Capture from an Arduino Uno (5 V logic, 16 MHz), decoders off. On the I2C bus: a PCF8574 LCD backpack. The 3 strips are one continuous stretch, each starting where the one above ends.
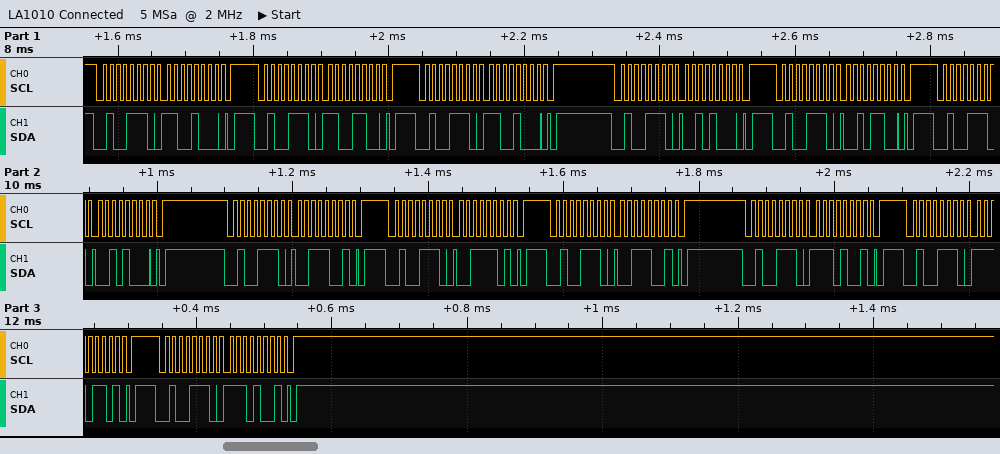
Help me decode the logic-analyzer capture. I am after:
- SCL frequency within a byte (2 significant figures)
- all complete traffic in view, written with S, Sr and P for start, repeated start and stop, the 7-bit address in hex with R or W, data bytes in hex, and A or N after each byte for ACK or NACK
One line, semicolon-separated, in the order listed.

100 kHz; S 27W A C8 A P S 27W A CC A P S 27W A C8 A P S 27W A 28 A P S 27W A 2C A P S 27W A 28 A P S 27W A 39 A P S 27W A 3D A P S 27W A 39 A P S 27W A E9 A P S 27W A ED A P S 27W A E9 A P
